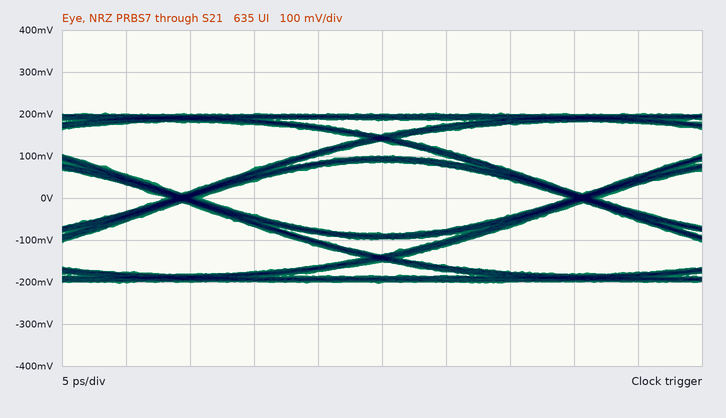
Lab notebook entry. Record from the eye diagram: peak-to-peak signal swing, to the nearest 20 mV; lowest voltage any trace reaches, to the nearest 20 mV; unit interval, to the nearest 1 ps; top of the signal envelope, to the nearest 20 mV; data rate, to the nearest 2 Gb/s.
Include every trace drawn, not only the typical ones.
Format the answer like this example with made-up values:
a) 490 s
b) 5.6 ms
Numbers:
a) 400 mV
b) -200 mV
c) 31 ps
d) 200 mV
e) 32 Gb/s
